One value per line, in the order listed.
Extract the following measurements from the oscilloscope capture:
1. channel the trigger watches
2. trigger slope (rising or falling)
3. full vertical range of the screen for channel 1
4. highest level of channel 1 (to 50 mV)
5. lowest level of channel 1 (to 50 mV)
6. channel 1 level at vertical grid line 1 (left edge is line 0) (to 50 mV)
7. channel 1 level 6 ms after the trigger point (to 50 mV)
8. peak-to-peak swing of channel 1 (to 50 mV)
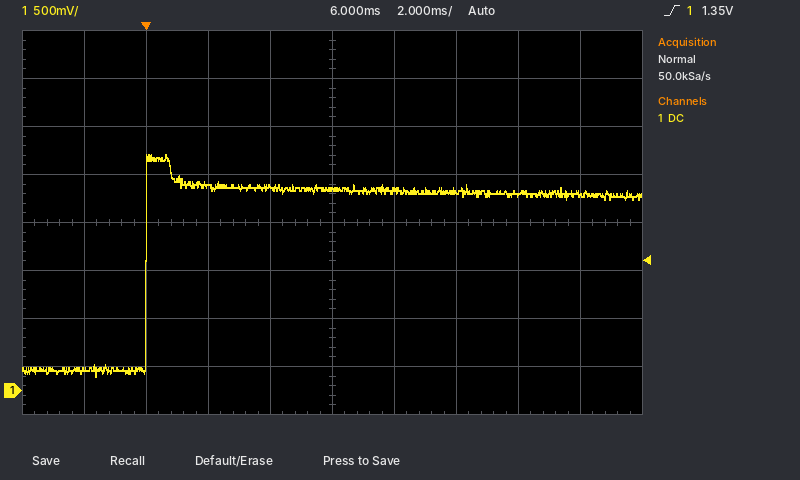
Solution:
channel 1
rising
4 V
2.45 V
150 mV
200 mV
2.10 V
2.30 V
